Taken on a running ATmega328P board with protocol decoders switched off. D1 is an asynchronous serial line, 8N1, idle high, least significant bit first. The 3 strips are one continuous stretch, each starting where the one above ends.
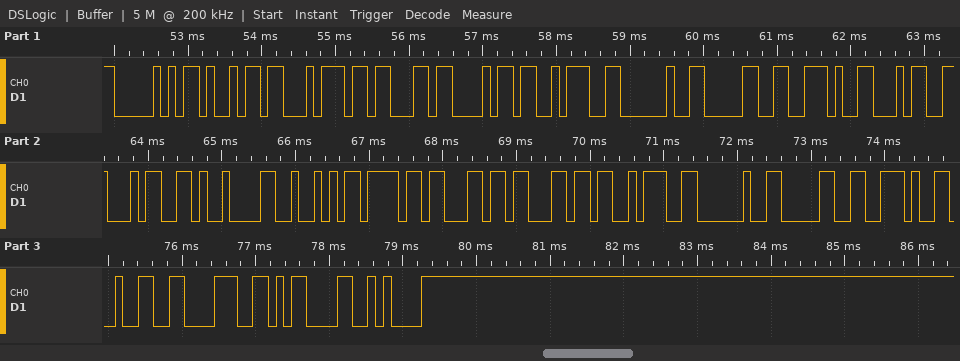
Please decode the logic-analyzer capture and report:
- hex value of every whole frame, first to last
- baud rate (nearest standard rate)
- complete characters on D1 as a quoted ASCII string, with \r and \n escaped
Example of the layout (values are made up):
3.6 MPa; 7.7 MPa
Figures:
50 69 74 63 68 3A 20 30 2E 34 34 09 52 6F 6C 6C 3A 20 30 2E 32 38 0D 0A; 9600 baud; "Pitch: 0.44\tRoll: 0.28\r\n"
